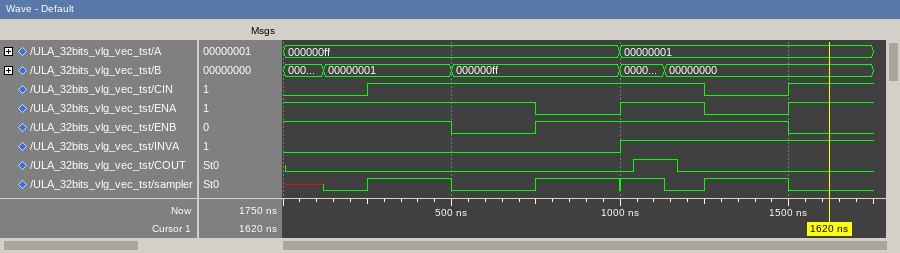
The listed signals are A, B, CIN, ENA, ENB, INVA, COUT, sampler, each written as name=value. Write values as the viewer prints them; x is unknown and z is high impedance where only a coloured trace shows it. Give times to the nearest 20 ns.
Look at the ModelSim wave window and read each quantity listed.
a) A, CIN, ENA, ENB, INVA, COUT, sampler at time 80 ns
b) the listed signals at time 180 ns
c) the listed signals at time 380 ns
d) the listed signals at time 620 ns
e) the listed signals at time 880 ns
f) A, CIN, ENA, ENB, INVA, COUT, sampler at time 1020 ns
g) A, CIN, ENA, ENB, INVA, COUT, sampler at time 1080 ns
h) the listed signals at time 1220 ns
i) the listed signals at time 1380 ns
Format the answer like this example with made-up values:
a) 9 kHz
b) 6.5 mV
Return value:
a) A=000000ff, CIN=0, ENA=1, ENB=1, INVA=0, COUT=0, sampler=x
b) A=000000ff, B=00000001, CIN=0, ENA=1, ENB=1, INVA=0, COUT=0, sampler=0
c) A=000000ff, B=00000001, CIN=1, ENA=1, ENB=1, INVA=0, COUT=0, sampler=1
d) A=000000ff, B=000000ff, CIN=1, ENA=1, ENB=0, INVA=0, COUT=0, sampler=0
e) A=000000ff, B=000000ff, CIN=1, ENA=0, ENB=1, INVA=0, COUT=0, sampler=1
f) A=00000001, CIN=1, ENA=1, ENB=1, INVA=1, COUT=0, sampler=1
g) A=00000001, CIN=1, ENA=1, ENB=1, INVA=1, COUT=1, sampler=1
h) A=00000001, B=00000000, CIN=1, ENA=1, ENB=1, INVA=1, COUT=0, sampler=0
i) A=00000001, B=00000000, CIN=0, ENA=0, ENB=1, INVA=1, COUT=0, sampler=1
